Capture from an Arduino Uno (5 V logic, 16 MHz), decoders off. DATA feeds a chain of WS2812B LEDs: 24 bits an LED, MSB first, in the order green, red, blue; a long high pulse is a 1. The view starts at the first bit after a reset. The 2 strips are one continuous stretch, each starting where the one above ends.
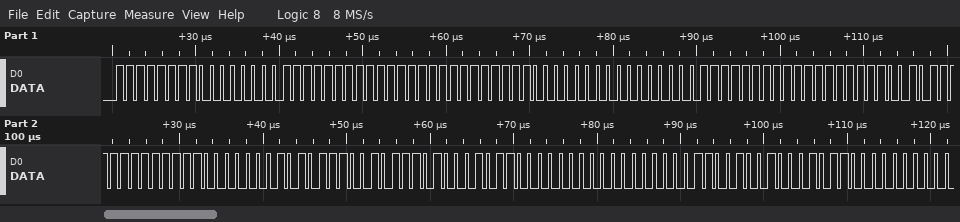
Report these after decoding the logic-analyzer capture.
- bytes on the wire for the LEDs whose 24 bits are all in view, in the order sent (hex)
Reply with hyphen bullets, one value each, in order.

- FF 00 FF FF FF 00 00 FF FF CB FF C0 57 2E 8B 00 00 64
